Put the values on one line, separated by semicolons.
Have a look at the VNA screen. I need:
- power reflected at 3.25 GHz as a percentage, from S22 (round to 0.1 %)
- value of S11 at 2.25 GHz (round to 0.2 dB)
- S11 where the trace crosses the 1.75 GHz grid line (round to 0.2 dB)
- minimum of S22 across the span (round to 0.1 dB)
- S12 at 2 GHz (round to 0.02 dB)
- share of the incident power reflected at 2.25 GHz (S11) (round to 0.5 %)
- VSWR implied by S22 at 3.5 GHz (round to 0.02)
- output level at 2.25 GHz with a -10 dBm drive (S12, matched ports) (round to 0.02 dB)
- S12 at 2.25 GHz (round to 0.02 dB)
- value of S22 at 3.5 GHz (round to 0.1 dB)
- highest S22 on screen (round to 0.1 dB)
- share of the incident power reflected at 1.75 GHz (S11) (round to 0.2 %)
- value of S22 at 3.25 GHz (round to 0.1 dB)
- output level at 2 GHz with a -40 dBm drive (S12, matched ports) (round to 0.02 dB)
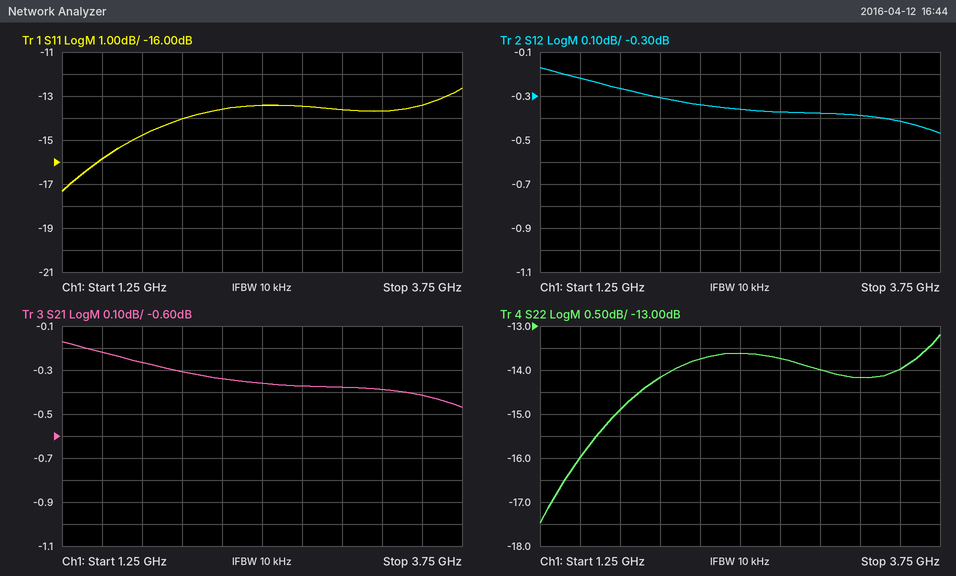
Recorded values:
3.8 %; -13.6 dB; -14.8 dB; -17.5 dB; -0.30 dB; 4.5 %; 1.50; -10.34 dBm; -0.34 dB; -14.0 dB; -13.2 dB; 3.4 %; -14.2 dB; -40.30 dBm
